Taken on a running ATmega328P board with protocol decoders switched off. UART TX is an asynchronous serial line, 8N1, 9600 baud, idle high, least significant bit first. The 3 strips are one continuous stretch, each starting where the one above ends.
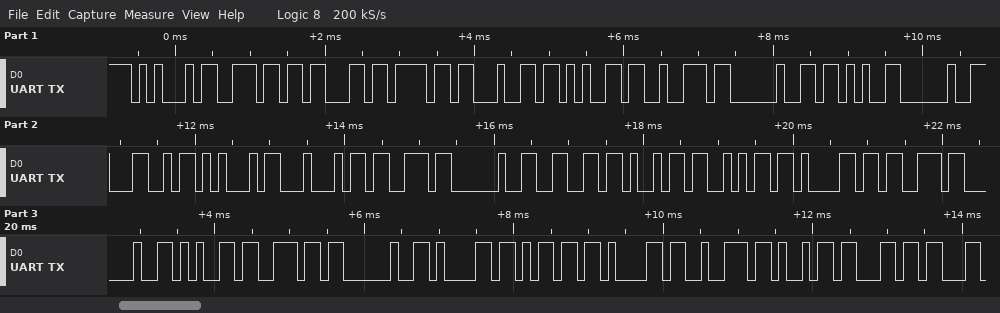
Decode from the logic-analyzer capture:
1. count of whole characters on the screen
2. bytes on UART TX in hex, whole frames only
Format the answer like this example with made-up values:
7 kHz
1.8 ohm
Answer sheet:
30
45 6E 63 6F 64 65 72 20 2B 20 4C 45 44 73 20 66 69 6A 61 73 20 65 6E 20 61 6D 61 72 69 6C
